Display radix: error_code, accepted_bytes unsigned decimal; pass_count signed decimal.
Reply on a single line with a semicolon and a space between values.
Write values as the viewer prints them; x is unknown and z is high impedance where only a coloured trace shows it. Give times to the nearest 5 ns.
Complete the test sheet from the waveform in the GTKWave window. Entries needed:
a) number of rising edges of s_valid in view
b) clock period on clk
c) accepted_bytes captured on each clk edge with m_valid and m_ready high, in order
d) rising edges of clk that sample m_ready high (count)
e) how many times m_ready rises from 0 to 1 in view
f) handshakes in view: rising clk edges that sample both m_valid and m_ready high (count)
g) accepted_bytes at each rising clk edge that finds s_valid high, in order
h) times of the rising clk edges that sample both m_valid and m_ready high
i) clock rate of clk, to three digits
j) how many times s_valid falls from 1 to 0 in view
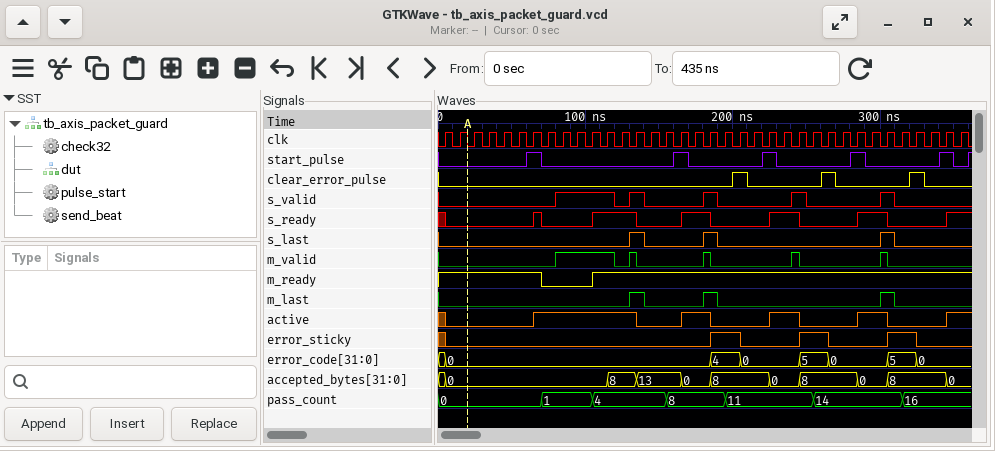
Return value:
5; 10 ns; 0, 8, 0, 0, 0; 32; 1; 5; 0, 0, 0, 0, 8, 0, 0, 0; 115 ns, 135 ns, 185 ns, 245 ns, 305 ns; 100 MHz; 5
